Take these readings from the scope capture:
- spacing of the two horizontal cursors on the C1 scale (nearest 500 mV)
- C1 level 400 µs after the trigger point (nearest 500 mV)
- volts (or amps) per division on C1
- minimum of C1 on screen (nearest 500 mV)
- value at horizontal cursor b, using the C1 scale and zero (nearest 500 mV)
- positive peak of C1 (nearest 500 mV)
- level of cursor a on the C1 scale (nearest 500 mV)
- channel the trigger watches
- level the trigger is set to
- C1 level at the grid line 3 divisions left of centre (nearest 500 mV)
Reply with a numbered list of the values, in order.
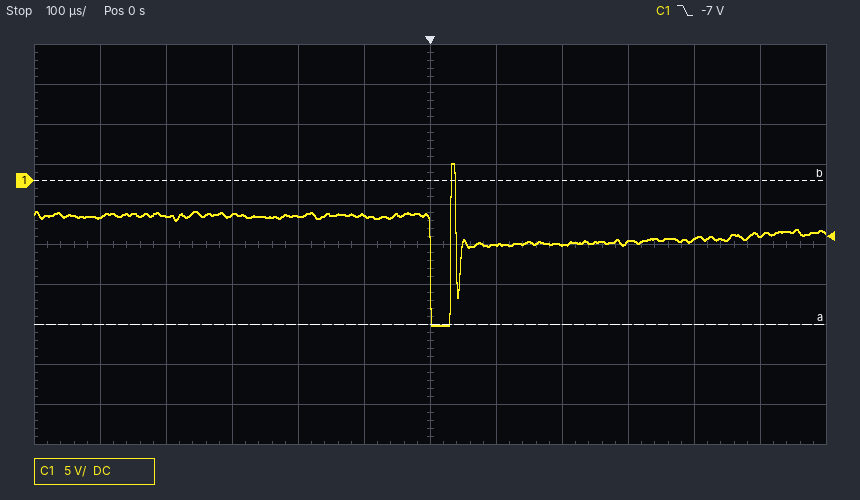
1. 18.0 V
2. -7.5 V
3. 5 V
4. -18.0 V
5. 0.0 V
6. 2.0 V
7. -18.0 V
8. C1
9. -7 V
10. -4.5 V
